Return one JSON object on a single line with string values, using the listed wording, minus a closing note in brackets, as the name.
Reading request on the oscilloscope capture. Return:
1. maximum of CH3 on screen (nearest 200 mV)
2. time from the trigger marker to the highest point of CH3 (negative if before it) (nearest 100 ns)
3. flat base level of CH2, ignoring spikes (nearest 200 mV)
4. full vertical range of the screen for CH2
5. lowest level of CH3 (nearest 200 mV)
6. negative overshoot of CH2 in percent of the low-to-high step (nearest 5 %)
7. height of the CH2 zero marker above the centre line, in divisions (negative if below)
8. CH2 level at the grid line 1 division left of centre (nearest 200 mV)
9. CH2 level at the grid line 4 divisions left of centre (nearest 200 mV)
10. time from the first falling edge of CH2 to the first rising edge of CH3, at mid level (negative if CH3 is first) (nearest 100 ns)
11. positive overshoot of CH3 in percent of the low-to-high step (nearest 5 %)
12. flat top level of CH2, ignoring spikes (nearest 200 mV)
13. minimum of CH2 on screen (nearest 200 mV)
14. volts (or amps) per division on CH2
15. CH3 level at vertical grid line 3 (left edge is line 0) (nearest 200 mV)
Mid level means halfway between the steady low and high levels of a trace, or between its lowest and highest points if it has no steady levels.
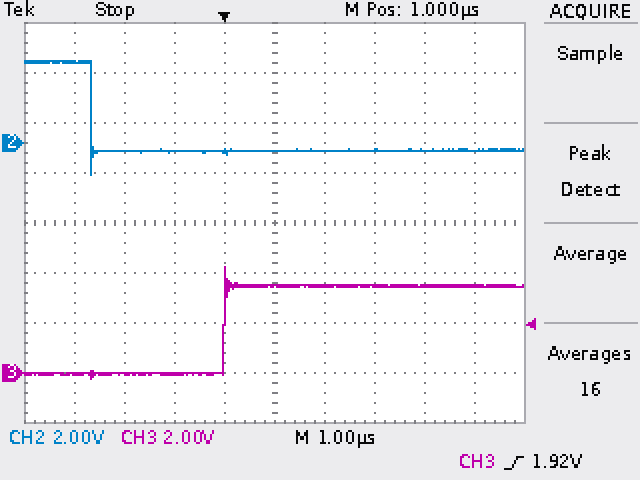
{"maximum of CH3 on screen": "4.2 V", "time from the trigger marker to the highest point of CH3 (negative if before it)": "0.0 µs", "flat base level of CH2, ignoring spikes": "-400 mV", "full vertical range of the screen for CH2": "16 V", "lowest level of CH3": "-200 mV", "negative overshoot of CH2 in percent of the low-to-high step": "25 %", "height of the CH2 zero marker above the centre line, in divisions": "+1.6 div", "CH2 level at the grid line 1 division left of centre": "-400 mV", "CH2 level at the grid line 4 divisions left of centre": "3.2 V", "time from the first falling edge of CH2 to the first rising edge of CH3, at mid level (negative if CH3 is first)": "+2.7 µs", "positive overshoot of CH3 in percent of the low-to-high step": "20 %", "flat top level of CH2, ignoring spikes": "3.2 V", "minimum of CH2 on screen": "-1.2 V", "volts (or amps) per division on CH2": "2 V", "CH3 level at vertical grid line 3 (left edge is line 0)": "0.0 V"}
